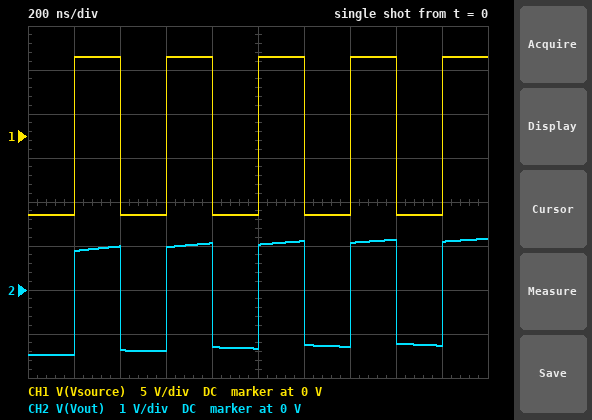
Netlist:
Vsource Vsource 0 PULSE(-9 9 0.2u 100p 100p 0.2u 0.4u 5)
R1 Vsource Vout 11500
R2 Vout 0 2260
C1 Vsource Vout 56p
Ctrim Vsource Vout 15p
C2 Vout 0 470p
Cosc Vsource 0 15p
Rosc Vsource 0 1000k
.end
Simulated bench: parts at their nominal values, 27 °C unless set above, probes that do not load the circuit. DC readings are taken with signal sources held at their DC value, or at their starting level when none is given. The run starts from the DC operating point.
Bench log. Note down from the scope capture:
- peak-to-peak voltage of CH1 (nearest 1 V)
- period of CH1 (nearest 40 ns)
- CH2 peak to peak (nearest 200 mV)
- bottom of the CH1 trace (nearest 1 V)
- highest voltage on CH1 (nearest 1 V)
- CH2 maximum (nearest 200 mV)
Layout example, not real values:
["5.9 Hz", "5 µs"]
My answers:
["18 V", "400 ns", "2.6 V", "-9 V", "9 V", "1.2 V"]
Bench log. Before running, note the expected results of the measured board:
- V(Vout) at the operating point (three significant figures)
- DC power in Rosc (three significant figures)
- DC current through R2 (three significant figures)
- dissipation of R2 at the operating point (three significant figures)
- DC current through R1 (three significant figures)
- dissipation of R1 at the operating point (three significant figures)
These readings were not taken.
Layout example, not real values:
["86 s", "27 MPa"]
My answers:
["-1.48 V", "81.0 µW", "654 µA", "967 µW", "654 µA", "4.92 mW"]
